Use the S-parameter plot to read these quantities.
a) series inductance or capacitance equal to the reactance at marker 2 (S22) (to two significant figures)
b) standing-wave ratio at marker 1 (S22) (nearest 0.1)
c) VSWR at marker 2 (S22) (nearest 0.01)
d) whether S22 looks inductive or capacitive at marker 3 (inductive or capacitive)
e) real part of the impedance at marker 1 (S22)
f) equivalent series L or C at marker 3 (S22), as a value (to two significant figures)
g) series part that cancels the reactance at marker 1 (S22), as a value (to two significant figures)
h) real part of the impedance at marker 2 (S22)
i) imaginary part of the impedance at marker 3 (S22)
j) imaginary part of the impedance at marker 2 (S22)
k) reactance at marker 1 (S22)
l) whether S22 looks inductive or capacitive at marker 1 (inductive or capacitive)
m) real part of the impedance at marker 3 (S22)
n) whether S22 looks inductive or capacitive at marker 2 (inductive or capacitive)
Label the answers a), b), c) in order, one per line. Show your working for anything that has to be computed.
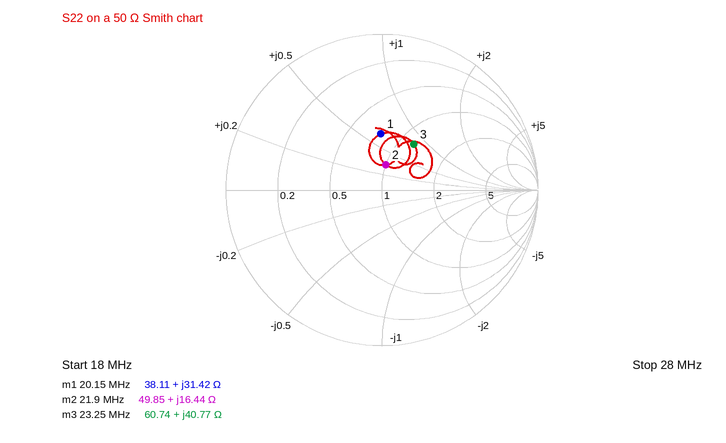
a) L = 16.44 Ω/(2π × 21.9 MHz) ≈ 119 nH, so 120 nH to two significant figures
b) 2.1
c) 1.39
d) inductive
e) 38.11 Ω
f) L = 40.77 Ω/(2π × 23.25 MHz) ≈ 279 nH, so 280 nH to two significant figures
g) C = 1/(2π × 20.15 MHz × 31.42 Ω) ≈ 251 pF, so 250 pF to two significant figures
h) 49.85 Ω
i) +40.77 Ω
j) +16.44 Ω
k) +31.42 Ω
l) inductive
m) 60.74 Ω
n) inductive
